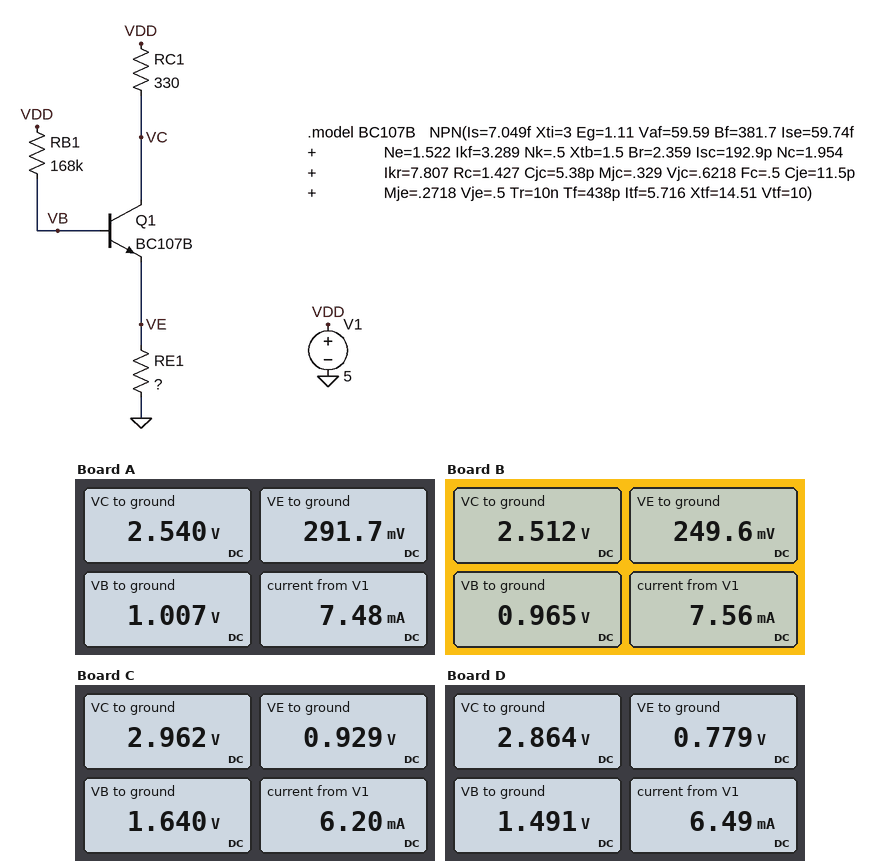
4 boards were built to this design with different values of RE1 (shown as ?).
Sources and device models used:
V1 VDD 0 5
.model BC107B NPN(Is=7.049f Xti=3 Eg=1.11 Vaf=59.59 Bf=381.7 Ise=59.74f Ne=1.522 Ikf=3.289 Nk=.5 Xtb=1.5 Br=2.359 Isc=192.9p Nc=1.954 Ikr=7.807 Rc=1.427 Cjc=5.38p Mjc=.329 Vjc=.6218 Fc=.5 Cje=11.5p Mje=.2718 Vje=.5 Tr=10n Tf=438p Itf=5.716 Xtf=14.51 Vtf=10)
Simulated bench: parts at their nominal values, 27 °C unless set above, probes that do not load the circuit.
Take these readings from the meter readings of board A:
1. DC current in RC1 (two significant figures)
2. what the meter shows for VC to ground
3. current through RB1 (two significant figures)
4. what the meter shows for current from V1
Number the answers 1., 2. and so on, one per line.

1. 7.5 mA
2. 2.540 V
3. 24 µA
4. 7.48 mA
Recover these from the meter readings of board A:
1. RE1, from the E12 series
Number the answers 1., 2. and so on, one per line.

1. 39 Ω
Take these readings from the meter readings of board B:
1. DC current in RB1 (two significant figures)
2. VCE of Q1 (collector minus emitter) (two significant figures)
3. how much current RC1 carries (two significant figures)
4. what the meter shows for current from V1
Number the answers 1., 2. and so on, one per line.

1. 24 µA
2. 2.3 V
3. 7.5 mA
4. 7.56 mA
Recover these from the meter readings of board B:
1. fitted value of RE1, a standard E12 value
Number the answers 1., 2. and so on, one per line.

1. 33 Ω
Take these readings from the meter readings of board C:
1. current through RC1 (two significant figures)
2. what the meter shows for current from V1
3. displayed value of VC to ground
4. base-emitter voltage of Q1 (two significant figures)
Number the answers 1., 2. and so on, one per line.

1. 6.2 mA
2. 6.20 mA
3. 2.962 V
4. 710 mV
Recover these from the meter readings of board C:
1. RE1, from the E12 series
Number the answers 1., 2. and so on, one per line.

1. 150 Ω
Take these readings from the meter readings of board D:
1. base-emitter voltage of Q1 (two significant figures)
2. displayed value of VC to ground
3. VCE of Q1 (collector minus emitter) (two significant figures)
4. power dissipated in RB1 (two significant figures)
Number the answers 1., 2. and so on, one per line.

1. 710 mV
2. 2.864 V
3. 2.1 V
4. 73 µW
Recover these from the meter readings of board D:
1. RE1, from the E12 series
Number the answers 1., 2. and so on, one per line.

1. 120 Ω
